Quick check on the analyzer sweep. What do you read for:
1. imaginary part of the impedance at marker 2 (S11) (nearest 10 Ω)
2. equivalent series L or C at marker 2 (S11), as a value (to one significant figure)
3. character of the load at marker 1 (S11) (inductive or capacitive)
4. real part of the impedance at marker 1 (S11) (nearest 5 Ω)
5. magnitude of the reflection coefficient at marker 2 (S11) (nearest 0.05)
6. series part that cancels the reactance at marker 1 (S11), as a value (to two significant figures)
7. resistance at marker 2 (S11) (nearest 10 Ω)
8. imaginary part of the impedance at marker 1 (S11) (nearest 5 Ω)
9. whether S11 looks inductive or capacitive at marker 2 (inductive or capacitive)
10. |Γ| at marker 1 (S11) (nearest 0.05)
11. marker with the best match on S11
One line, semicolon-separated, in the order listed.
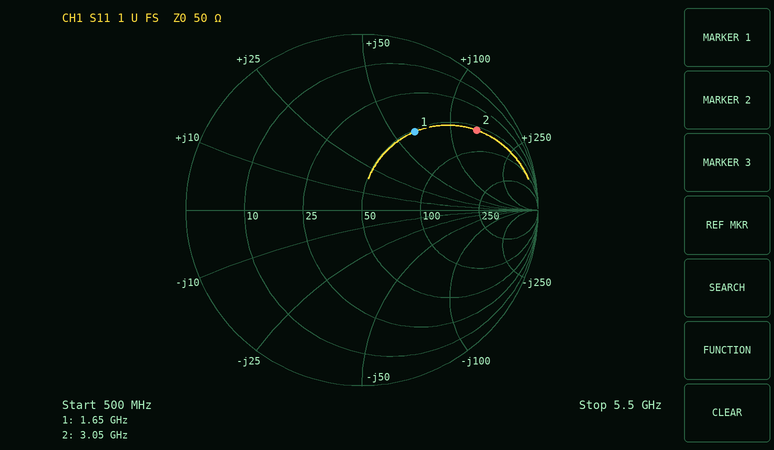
+140 Ω; 7 nH; inductive; 50 Ω; 0.80; 1.5 pF; 60 Ω; +65 Ω; inductive; 0.55; marker 1
